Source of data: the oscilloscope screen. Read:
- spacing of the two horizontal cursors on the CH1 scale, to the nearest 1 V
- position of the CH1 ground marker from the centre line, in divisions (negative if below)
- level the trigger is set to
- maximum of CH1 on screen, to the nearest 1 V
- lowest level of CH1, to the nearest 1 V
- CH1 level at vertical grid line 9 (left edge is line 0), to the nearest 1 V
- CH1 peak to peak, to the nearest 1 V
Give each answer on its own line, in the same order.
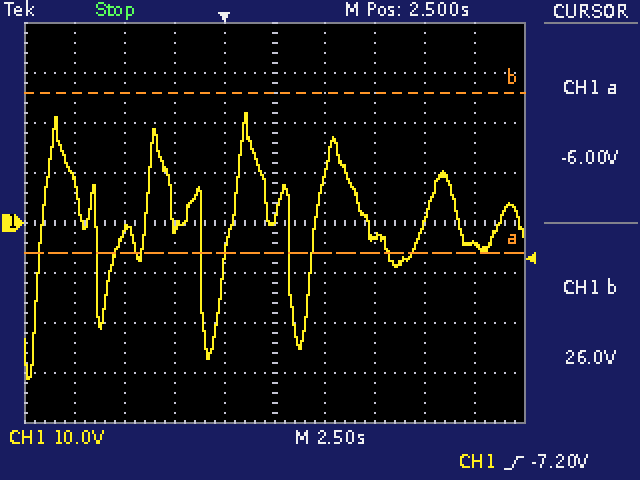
32 V
0.0 div
-7.20 V
22 V
-31 V
-4 V
53 V
